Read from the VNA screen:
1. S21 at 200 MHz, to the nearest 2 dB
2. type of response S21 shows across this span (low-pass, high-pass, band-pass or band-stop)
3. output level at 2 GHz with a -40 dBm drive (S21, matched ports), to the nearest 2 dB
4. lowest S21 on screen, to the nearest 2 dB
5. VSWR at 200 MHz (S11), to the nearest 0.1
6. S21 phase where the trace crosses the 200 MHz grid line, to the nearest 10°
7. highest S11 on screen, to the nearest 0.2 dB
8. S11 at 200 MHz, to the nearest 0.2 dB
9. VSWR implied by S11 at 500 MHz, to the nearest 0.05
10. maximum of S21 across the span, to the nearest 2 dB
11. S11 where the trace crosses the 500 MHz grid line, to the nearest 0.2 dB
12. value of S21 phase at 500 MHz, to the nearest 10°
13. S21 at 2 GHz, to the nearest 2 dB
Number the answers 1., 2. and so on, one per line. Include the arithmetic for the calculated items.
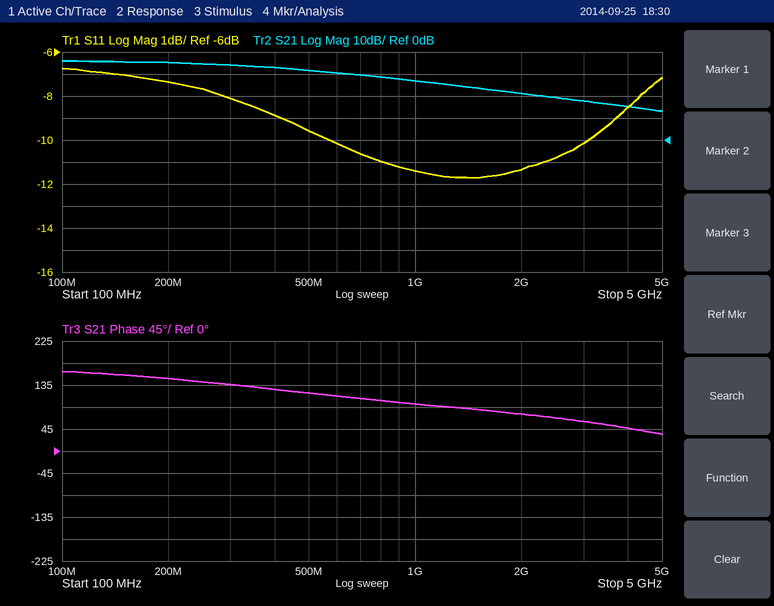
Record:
1. 36 dB
2. low-pass
3. -40 dBm + (22 dB) = -18 dBm
4. 14 dB
5. |Γ| = 10^(-7.4/20) = 0.4266; VSWR = (1 + 0.4266)/(1 − 0.4266) ≈ 2.5
6. 150°
7. -6.8 dB
8. -7.4 dB
9. |Γ| = 10^(-9.6/20) = 0.3311; VSWR = (1 + 0.3311)/(1 − 0.3311) ≈ 1.99, so 2.00 to the nearest 0.05
10. 36 dB
11. -9.6 dB
12. 120°
13. 22 dB
